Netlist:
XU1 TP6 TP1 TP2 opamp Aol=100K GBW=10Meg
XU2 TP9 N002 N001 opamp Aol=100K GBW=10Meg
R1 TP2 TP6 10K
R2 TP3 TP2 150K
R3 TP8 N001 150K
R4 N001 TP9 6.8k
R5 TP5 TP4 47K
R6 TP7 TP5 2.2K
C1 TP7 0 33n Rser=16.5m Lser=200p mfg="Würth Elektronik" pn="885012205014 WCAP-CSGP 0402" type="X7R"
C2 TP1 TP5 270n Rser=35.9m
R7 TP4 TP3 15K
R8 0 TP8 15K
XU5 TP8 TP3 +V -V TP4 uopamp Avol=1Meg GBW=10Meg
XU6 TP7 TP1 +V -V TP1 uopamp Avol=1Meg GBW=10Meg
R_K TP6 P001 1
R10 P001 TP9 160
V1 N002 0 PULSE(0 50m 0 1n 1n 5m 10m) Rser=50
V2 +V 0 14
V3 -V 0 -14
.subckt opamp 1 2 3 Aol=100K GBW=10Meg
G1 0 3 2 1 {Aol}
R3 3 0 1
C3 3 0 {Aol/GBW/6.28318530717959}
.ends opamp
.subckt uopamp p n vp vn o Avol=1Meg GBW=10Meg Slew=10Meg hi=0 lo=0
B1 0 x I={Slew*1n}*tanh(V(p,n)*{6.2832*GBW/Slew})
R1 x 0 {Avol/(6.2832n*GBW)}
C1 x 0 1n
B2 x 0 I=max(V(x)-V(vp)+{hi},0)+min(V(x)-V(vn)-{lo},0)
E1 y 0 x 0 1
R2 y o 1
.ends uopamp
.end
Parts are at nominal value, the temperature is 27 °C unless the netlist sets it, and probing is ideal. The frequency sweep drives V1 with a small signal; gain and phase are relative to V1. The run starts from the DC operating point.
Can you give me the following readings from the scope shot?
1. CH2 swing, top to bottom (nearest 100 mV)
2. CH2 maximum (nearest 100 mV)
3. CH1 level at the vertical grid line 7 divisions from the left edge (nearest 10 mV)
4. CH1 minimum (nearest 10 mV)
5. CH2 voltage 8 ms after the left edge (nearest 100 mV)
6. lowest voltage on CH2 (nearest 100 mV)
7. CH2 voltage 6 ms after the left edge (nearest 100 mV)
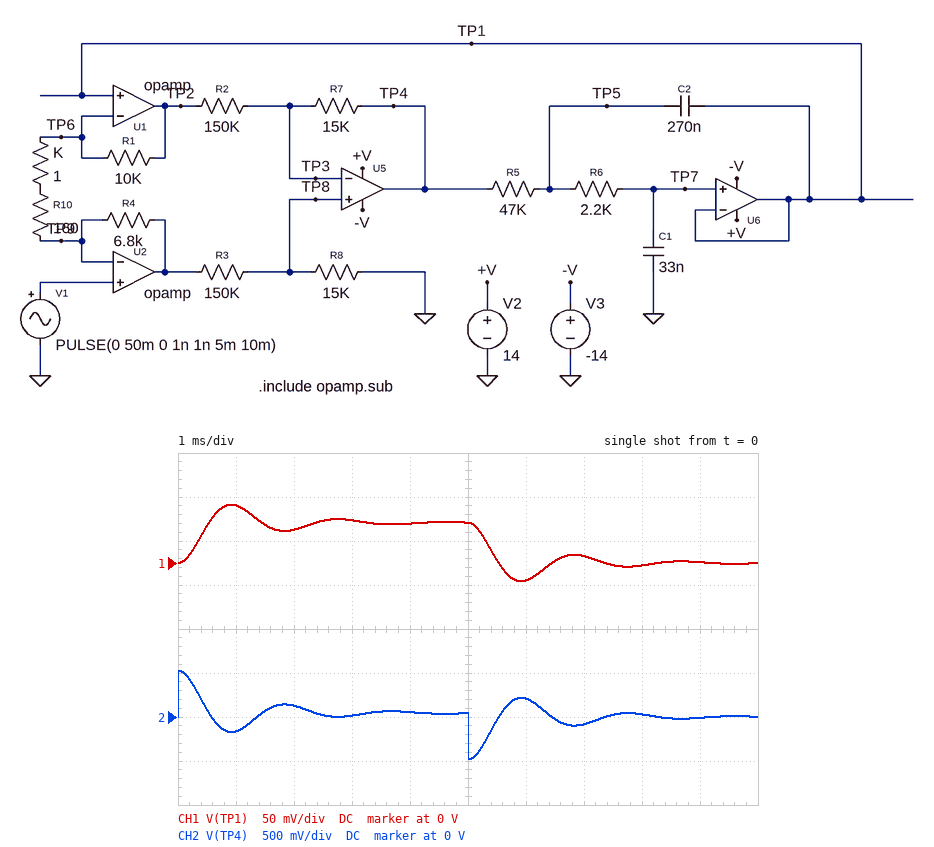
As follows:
1.0 V
500 mV
10 mV
-20 mV
0 V
-500 mV
200 mV
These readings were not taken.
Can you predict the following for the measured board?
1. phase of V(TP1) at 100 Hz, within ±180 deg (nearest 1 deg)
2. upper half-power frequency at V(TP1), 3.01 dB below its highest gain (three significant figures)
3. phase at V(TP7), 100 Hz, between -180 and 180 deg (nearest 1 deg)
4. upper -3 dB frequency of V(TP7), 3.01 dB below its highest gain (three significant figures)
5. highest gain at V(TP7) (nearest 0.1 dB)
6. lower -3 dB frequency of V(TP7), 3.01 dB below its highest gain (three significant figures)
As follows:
-5 deg
655 Hz
-5 deg
655 Hz
5.6 dB
356 Hz
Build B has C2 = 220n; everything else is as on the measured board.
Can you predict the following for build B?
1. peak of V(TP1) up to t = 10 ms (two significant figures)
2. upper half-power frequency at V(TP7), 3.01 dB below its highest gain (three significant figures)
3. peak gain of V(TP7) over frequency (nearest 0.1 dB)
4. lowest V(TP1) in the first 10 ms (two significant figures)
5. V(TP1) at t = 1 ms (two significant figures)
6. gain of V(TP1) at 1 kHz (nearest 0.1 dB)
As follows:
64 mV
731 Hz
4.8 dB
-19 mV
61 mV
-5.9 dB
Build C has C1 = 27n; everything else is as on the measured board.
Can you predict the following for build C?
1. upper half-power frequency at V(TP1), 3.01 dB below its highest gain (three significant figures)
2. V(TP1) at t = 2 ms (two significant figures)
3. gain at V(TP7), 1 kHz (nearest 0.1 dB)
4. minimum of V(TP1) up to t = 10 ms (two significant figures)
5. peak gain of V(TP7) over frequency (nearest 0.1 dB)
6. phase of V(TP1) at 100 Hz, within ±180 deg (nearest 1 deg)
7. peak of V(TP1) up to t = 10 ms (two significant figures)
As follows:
719 Hz
42 mV
-5.6 dB
-22 mV
6.5 dB
-4 deg
68 mV
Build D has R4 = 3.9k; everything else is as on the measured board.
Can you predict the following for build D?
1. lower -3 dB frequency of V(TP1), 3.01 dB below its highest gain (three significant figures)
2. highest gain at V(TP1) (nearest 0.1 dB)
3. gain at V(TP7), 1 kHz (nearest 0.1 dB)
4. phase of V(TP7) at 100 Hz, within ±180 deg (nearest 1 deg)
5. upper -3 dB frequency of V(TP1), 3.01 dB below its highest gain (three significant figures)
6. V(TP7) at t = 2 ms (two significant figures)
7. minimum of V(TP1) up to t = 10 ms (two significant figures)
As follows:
300 Hz
4.8 dB
-10.3 dB
-6 deg
606 Hz
37 mV
-19 mV
